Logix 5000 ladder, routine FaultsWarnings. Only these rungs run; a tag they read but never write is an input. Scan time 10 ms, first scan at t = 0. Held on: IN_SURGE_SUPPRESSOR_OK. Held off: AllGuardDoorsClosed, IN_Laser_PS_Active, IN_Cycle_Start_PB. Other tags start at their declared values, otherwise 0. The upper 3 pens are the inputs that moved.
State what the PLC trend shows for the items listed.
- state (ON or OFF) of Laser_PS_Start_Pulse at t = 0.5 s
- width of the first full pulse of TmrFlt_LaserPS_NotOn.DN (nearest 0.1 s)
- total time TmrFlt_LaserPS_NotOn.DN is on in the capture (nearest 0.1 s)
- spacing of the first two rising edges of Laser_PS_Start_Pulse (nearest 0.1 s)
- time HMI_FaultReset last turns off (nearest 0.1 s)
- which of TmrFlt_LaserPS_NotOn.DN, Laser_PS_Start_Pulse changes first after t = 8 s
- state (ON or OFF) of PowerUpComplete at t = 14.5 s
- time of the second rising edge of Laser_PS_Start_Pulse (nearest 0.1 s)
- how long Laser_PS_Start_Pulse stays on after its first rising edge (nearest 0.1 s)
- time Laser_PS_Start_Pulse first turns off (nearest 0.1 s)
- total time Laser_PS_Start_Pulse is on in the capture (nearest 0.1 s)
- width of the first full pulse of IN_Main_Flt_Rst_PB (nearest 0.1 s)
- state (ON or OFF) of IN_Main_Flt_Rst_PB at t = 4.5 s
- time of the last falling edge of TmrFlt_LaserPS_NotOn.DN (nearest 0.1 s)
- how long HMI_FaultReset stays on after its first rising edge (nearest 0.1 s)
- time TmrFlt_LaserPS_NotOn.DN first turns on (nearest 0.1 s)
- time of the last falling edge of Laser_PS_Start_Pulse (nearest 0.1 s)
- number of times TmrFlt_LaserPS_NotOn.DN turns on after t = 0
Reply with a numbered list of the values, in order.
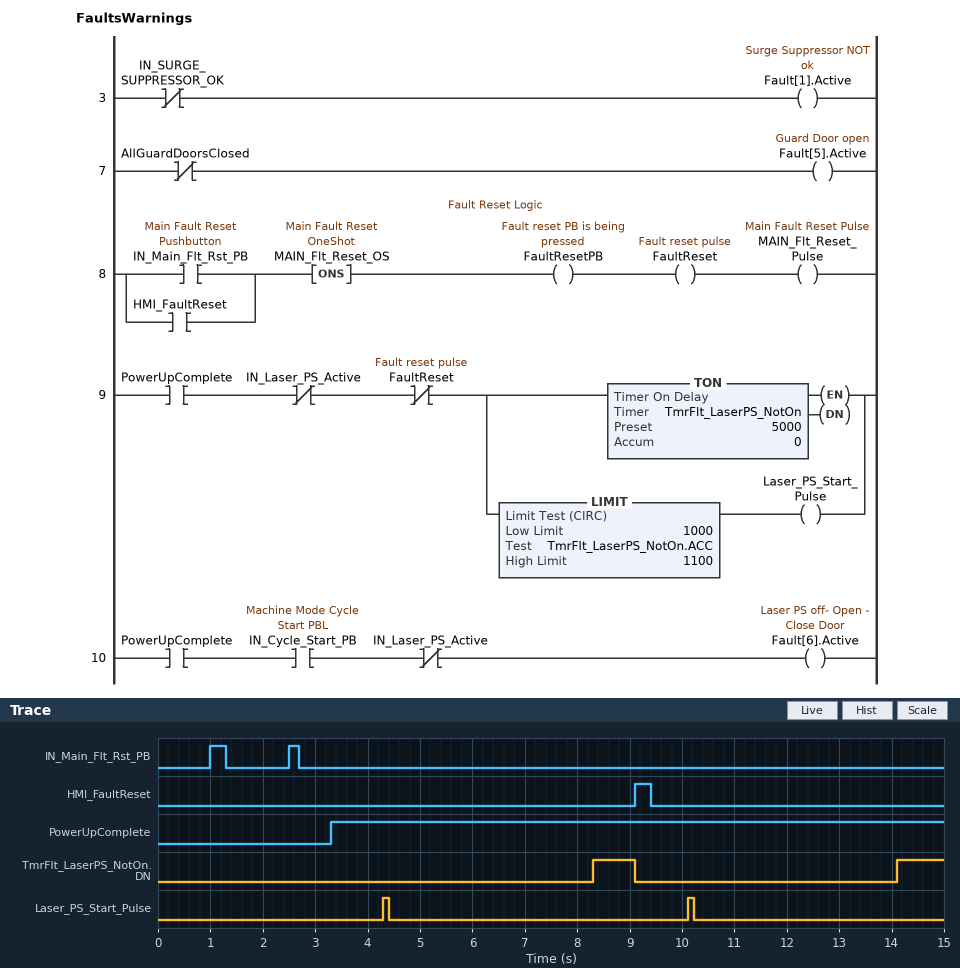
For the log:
1. OFF
2. 0.8 s
3. 1.7 s
4. 5.8 s
5. 9.4 s
6. TmrFlt_LaserPS_NotOn.DN
7. ON
8. 10.1 s
9. 0.1 s
10. 4.4 s
11. 0.2 s
12. 0.3 s
13. OFF
14. 9.1 s
15. 0.3 s
16. 8.3 s
17. 10.2 s
18. 2
